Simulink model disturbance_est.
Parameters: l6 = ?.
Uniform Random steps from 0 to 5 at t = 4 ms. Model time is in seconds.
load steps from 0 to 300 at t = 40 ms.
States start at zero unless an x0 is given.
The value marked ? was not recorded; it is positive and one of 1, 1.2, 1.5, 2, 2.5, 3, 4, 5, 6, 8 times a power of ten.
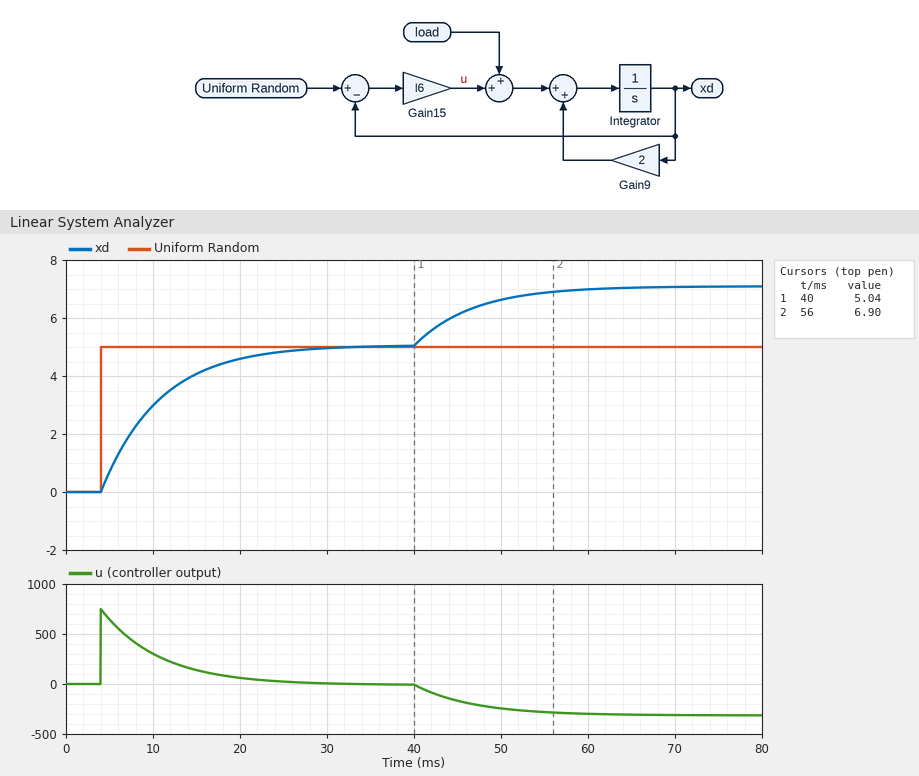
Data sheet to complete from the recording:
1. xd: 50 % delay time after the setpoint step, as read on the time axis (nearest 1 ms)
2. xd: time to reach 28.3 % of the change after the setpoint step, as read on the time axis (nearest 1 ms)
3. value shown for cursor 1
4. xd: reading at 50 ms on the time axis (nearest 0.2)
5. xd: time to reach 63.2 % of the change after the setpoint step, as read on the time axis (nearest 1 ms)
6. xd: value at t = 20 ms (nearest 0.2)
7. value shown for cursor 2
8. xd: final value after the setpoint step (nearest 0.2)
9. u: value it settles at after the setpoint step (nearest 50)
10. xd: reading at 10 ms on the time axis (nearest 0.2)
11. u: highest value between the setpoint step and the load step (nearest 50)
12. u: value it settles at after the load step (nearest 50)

9 ms
6 ms
5.04
6.6
11 ms
4.6
6.90
5.0
0
3.0
750
-300
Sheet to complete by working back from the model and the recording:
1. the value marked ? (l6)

150
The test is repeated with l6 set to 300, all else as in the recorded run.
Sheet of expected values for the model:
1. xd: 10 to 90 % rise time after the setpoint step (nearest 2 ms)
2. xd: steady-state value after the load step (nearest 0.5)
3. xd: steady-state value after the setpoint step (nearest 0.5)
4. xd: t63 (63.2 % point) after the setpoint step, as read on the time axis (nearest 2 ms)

8 ms
6.0
5.0
8 ms
